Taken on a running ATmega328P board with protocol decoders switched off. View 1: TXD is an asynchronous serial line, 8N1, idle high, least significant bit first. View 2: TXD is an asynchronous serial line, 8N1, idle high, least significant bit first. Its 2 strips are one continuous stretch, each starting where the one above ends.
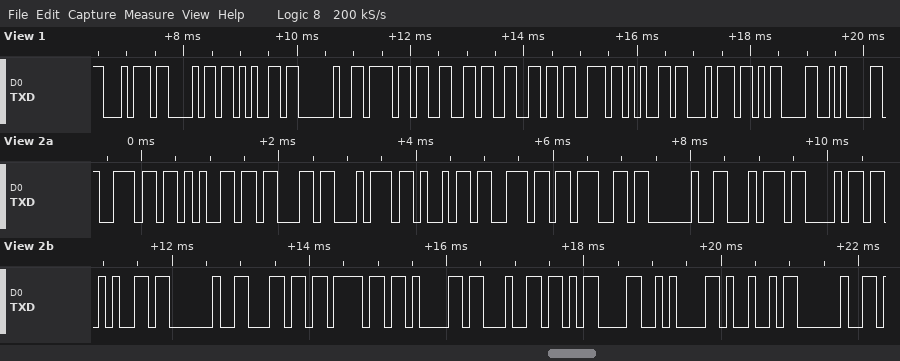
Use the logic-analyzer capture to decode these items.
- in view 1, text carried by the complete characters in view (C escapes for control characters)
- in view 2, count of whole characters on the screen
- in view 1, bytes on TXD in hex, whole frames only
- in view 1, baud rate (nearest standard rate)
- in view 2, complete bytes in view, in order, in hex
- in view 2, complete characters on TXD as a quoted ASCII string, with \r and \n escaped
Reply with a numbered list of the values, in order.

1. "the offset\r\n"
2. 20
3. 0x74 0x68 0x65 0x20 0x6F 0x66 0x66 0x73 0x65 0x74 0x0D 0x0A
4. 9600 baud
5. 6E 65 63 74 69 6E 67 20 74 68 65 20 6C 6F 61 64 0D 0A 49 20
6. "necting the load\r\nI "
